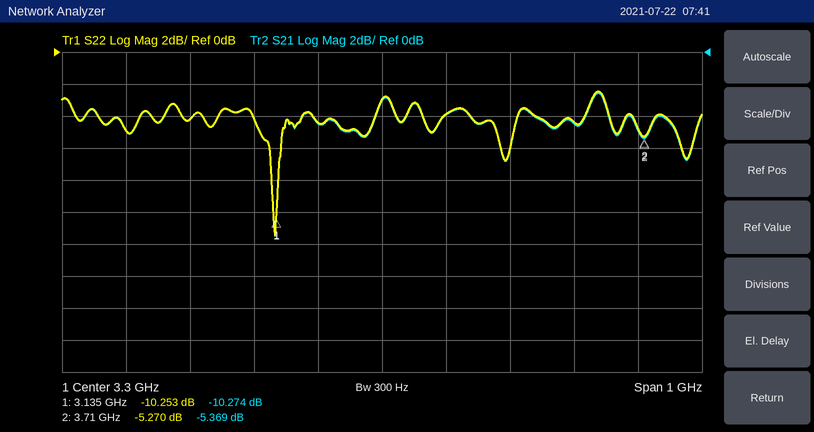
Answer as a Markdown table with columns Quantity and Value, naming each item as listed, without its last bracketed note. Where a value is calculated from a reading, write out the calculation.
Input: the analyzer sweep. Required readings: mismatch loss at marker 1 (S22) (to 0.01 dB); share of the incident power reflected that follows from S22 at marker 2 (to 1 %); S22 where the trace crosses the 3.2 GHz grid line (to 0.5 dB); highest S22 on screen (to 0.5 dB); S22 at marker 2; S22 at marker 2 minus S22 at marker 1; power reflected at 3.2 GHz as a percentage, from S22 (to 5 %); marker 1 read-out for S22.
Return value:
| Quantity | Value |
|---|---|
| mismatch loss at marker 1 (S22) | −10 log10(1 − 10^(-10.253/10)) ≈ 0.43 dB |
| share of the incident power reflected that follows from S22 at marker 2 | 10^(-5.27/10) ≈ 30 % |
| S22 where the trace crosses the 3.2 GHz grid line | -4.5 dB |
| highest S22 on screen | -2.5 dB |
| S22 at marker 2 | -5.270 dB |
| S22 at marker 2 minus S22 at marker 1 | -5.27 − (-10.253) = 4.983 dB |
| power reflected at 3.2 GHz as a percentage, from S22 | 10^(-4.5/10) ≈ 35 % |
| marker 1 read-out for S22 | -10.253 dB |
